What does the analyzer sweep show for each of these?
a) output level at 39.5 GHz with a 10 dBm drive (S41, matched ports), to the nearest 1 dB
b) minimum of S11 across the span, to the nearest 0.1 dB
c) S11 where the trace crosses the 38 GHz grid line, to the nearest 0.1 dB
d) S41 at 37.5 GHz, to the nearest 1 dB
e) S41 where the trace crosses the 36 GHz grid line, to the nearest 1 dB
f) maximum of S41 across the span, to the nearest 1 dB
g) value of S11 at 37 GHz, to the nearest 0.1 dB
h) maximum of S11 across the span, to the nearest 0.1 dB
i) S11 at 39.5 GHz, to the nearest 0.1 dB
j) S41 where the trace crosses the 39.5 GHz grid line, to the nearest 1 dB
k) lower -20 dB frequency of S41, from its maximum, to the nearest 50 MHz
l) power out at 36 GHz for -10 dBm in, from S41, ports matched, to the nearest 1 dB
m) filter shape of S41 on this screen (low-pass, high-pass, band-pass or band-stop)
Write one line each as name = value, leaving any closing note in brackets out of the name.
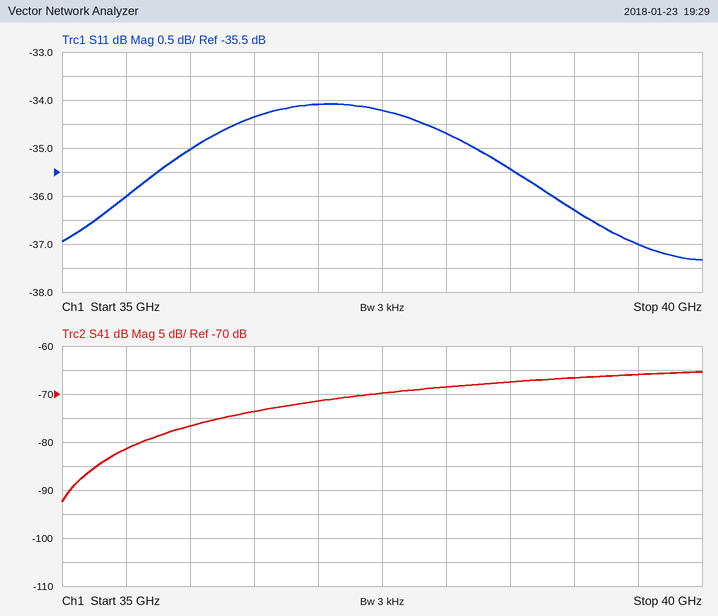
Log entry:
output level at 39.5 GHz with a 10 dBm drive (S41, matched ports), to the nearest 1 dB = -56 dBm
minimum of S11 across the span, to the nearest 0.1 dB = -37.3 dB
S11 where the trace crosses the 38 GHz grid line, to the nearest 0.1 dB = -34.7 dB
S41 at 37.5 GHz, to the nearest 1 dB = -70 dB
S41 where the trace crosses the 36 GHz grid line, to the nearest 1 dB = -77 dB
maximum of S41 across the span, to the nearest 1 dB = -65 dB
value of S11 at 37 GHz, to the nearest 0.1 dB = -34.1 dB
maximum of S11 across the span, to the nearest 0.1 dB = -34.1 dB
S11 at 39.5 GHz, to the nearest 0.1 dB = -37.0 dB
S41 where the trace crosses the 39.5 GHz grid line, to the nearest 1 dB = -66 dB
lower -20 dB frequency of S41, from its maximum, to the nearest 50 MHz = 35.25 GHz
power out at 36 GHz for -10 dBm in, from S41, ports matched, to the nearest 1 dB = -87 dBm
filter shape of S41 on this screen = high-pass
